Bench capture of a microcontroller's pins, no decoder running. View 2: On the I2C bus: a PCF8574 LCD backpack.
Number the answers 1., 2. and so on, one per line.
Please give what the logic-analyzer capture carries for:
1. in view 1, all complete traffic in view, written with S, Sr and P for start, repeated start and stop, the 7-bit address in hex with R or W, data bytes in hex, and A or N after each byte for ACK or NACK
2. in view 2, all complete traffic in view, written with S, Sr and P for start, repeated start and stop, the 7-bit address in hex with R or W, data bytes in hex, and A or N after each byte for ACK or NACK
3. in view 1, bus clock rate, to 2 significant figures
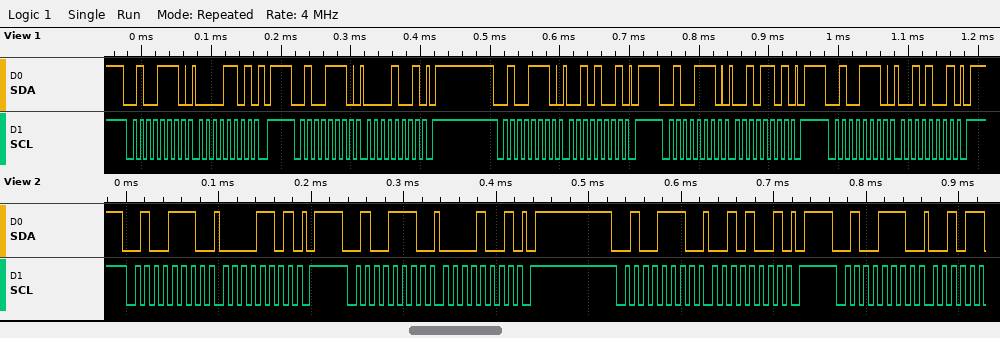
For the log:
1. S 27W A 0D A P S 27W A 09 A P S 27W A 29 A P S 27W A 2D A P S 27W A 29 A P
2. S 27W A 0D A P S 27W A 09 A P S 27W A 29 A P S 27W A
3. 100 kHz
